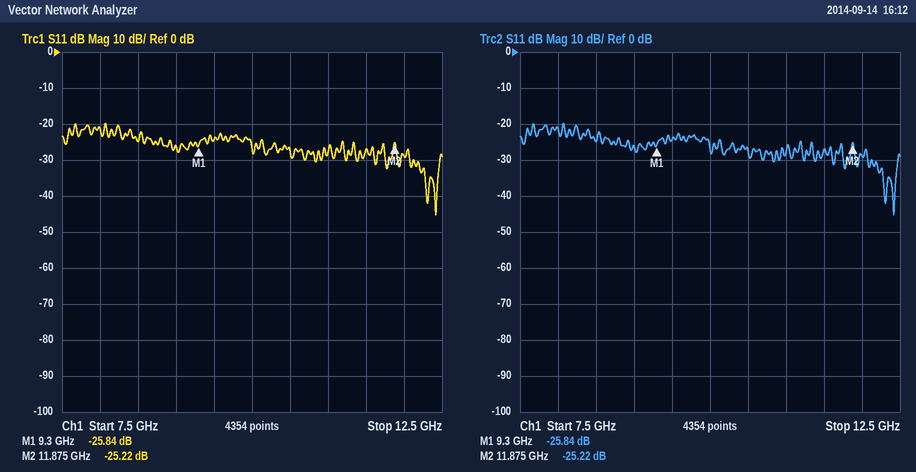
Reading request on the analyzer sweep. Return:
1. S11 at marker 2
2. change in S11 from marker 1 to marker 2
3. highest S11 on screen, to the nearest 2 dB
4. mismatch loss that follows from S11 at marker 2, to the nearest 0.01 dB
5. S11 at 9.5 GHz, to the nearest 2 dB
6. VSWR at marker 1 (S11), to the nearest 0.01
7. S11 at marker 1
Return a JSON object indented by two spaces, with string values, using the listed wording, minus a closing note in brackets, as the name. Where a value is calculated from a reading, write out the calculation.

{
  "S11 at marker 2": "-25.22 dB",
  "change in S11 from marker 1 to marker 2": "-25.22 − (-25.84) = 0.62 dB",
  "highest S11 on screen, to the nearest 2 dB": "-20 dB",
  "mismatch loss that follows from S11 at marker 2, to the nearest 0.01 dB": "−10 log10(1 − 10^(-25.22/10)) ≈ 0.01 dB",
  "S11 at 9.5 GHz, to the nearest 2 dB": "-24 dB",
  "VSWR at marker 1 (S11), to the nearest 0.01": "(1 + 0.0511)/(1 − 0.0511) ≈ 1.11",
  "S11 at marker 1": "-25.84 dB"
}
